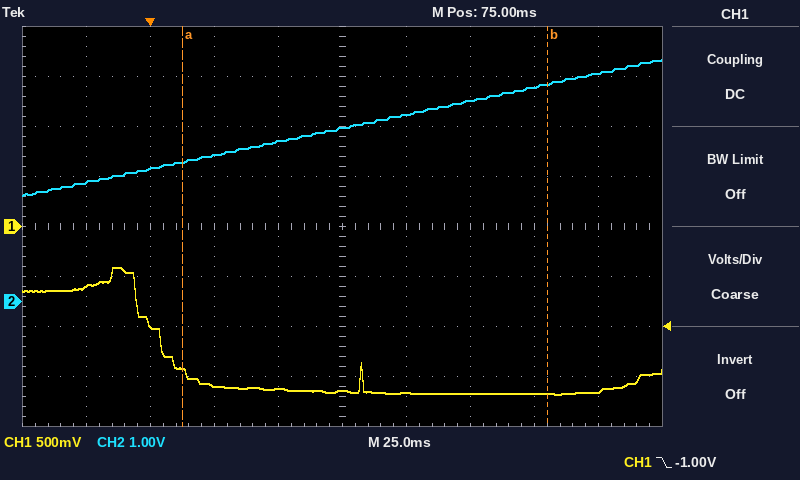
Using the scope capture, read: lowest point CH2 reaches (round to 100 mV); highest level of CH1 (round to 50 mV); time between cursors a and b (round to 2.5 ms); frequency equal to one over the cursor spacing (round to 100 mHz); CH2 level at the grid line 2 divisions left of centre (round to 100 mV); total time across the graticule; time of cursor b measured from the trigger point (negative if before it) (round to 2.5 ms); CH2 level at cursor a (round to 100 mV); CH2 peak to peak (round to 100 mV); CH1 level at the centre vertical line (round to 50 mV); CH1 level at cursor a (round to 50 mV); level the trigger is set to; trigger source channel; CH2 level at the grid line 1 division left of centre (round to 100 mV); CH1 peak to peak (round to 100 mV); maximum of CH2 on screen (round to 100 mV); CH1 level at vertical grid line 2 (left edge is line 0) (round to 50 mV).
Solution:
2.1 V
-400 mV
142.5 ms
7.0 Hz
2.9 V
250 ms
+155.0 ms
2.8 V
2.7 V
-1.65 V
-1.45 V
-1.00 V
CH1
3.2 V
1.30 V
4.8 V
-950 mV
